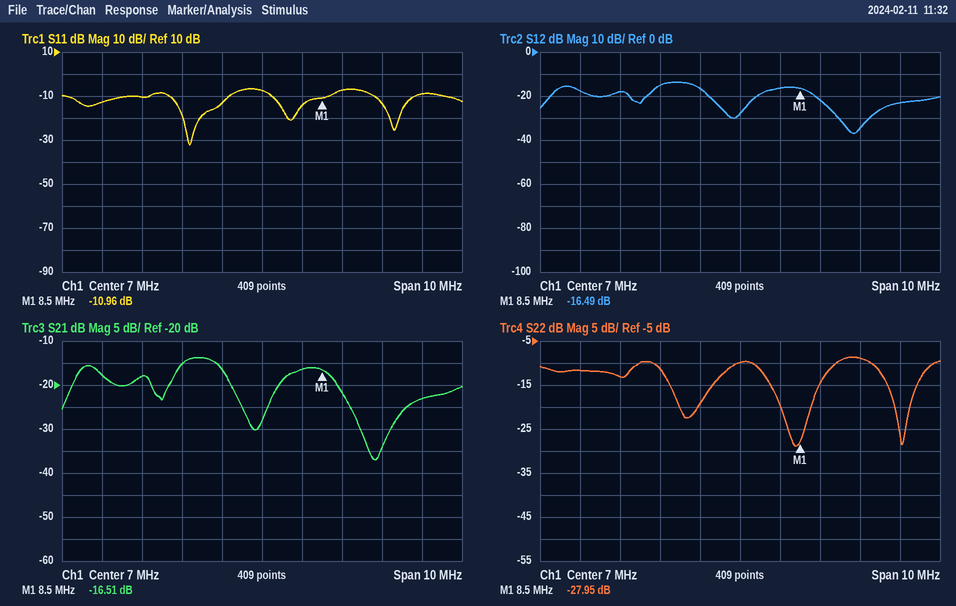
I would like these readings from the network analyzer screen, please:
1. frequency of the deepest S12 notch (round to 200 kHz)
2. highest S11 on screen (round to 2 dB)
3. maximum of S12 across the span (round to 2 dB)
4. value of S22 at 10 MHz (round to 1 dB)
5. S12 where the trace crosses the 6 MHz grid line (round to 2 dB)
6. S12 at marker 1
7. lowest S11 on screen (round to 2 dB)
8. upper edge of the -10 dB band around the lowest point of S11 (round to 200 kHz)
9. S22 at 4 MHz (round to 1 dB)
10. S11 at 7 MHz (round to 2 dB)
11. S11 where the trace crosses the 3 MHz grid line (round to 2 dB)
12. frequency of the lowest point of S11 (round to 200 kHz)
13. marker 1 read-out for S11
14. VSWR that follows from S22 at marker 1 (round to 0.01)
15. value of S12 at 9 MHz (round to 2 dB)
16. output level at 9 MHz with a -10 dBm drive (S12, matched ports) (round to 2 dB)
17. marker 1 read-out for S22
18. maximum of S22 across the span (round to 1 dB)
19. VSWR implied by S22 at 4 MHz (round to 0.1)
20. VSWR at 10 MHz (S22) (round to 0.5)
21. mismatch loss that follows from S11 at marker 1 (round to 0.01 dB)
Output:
9.8 MHz
-6 dB
-14 dB
-9 dB
-16 dB
-16.49 dB
-32 dB
6.2 MHz
-13 dB
-8 dB
-12 dB
5.2 MHz
-10.96 dB
1.08
-22 dB
-32 dBm
-27.95 dB
-9 dB
1.6
2.0
0.36 dB
